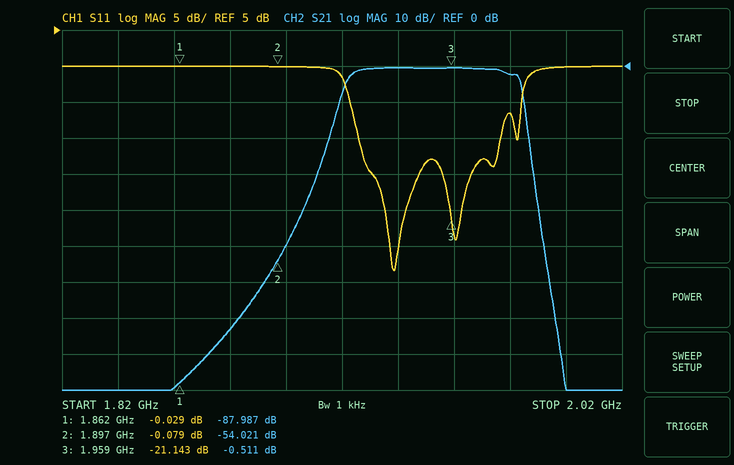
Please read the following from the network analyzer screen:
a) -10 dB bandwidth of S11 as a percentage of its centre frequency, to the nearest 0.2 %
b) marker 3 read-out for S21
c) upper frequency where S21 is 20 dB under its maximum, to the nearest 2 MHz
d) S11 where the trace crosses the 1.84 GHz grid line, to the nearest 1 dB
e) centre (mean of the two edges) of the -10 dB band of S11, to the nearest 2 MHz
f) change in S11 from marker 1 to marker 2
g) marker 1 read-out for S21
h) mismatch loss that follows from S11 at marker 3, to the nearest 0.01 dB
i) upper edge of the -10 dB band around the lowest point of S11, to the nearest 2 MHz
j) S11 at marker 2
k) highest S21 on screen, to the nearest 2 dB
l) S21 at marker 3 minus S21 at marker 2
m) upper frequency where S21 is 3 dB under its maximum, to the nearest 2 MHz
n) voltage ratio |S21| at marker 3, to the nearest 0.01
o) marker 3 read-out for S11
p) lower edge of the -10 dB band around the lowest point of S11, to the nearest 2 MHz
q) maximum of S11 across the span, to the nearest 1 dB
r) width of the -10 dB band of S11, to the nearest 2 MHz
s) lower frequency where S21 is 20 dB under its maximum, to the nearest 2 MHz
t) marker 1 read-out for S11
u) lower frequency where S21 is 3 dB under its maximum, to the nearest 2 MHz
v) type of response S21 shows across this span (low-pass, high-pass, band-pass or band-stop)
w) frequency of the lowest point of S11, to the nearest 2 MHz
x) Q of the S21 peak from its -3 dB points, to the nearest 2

2.6 %
-0.511 dB
1.986 GHz
0 dB
1.952 GHz
-0.050 dB
-87.987 dB
0.03 dB
1.976 GHz
-0.079 dB
0 dB
53.510 dB
1.984 GHz
0.94
-21.143 dB
1.926 GHz
0 dB
50 MHz
1.916 GHz
-0.029 dB
1.922 GHz
band-pass
1.938 GHz
32
